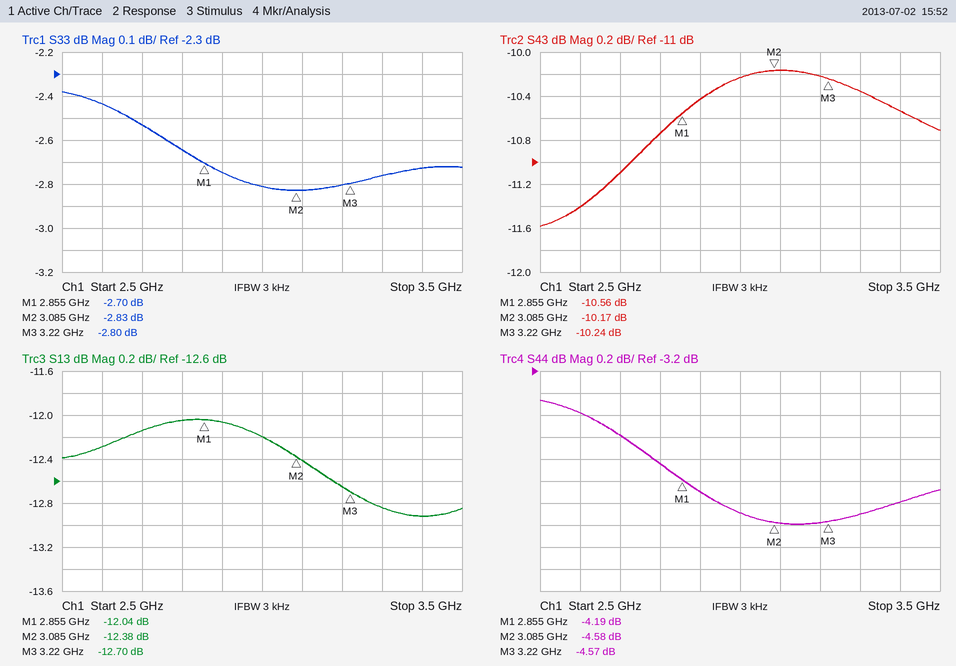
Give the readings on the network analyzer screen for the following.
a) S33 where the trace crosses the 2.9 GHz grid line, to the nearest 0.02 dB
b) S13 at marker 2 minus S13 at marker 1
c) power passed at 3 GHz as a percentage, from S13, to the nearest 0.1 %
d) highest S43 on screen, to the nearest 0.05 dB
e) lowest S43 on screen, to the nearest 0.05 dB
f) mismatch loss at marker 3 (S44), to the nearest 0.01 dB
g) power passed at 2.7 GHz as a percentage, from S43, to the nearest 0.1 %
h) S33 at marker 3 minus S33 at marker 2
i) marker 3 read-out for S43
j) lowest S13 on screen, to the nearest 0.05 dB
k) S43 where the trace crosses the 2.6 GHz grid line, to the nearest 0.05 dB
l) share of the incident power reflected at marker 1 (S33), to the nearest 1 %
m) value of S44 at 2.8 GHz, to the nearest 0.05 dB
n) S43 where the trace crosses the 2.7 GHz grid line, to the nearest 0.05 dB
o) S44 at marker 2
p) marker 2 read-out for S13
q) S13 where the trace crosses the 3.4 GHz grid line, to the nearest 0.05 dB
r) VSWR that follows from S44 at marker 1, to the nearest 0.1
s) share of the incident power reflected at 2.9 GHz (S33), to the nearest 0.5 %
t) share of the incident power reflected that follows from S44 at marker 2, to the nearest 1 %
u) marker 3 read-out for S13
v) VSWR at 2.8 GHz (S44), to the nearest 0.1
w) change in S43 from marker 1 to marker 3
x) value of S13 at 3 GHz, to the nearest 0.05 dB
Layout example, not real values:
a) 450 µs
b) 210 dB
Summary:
a) -2.74 dB
b) -0.34 dB
c) 6.0 %
d) -10.15 dB
e) -11.60 dB
f) 1.87 dB
g) 7.8 %
h) 0.03 dB
i) -10.24 dB
j) -12.90 dB
k) -11.40 dB
l) 54 %
m) -4.05 dB
n) -11.10 dB
o) -4.58 dB
p) -12.38 dB
q) -12.90 dB
r) 4.2
s) 53.0 %
t) 35 %
u) -12.70 dB
v) 4.4
w) 0.32 dB
x) -12.20 dB
